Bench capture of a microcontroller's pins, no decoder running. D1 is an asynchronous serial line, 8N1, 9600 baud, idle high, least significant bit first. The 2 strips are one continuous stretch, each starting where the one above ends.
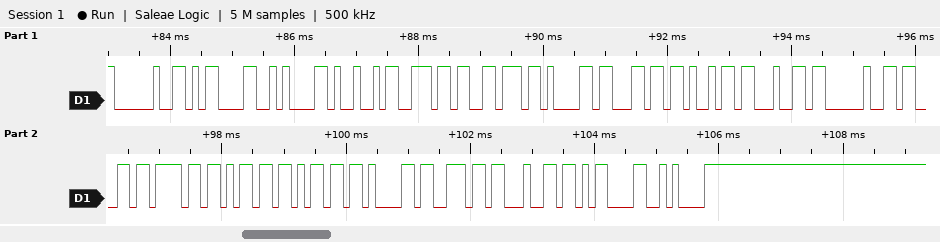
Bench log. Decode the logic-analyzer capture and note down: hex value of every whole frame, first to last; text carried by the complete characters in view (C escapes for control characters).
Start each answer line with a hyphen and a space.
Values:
- 20 0D 0A 49 6E 76 61 6C 69 64 20 63 6F 6D 6D 61 6E 64 0D 0A
- " \r\nInvalid command\r\n"
